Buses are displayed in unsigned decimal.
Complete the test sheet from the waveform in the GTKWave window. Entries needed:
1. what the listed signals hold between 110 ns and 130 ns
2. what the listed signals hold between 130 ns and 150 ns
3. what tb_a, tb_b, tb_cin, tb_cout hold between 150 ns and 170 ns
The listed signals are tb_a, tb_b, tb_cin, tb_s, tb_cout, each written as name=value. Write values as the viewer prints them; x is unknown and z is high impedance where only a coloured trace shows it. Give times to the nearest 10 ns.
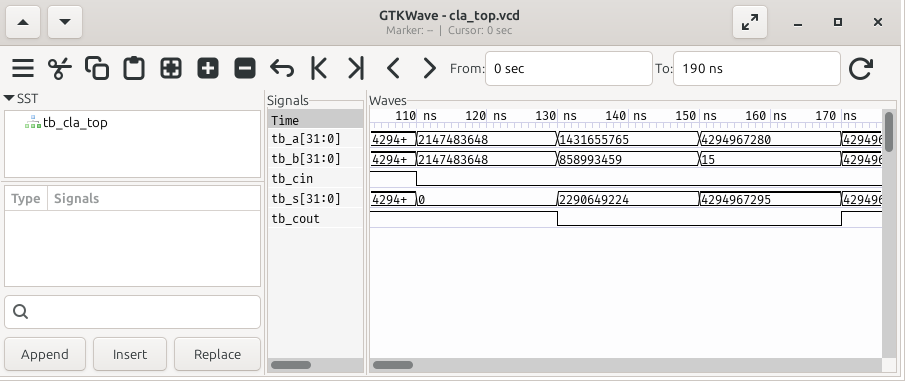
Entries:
tb_a=2147483648, tb_b=2147483648, tb_cin=0, tb_s=0, tb_cout=1
tb_a=1431655765, tb_b=858993459, tb_cin=0, tb_s=2290649224, tb_cout=0
tb_a=4294967280, tb_b=15, tb_cin=0, tb_cout=0
